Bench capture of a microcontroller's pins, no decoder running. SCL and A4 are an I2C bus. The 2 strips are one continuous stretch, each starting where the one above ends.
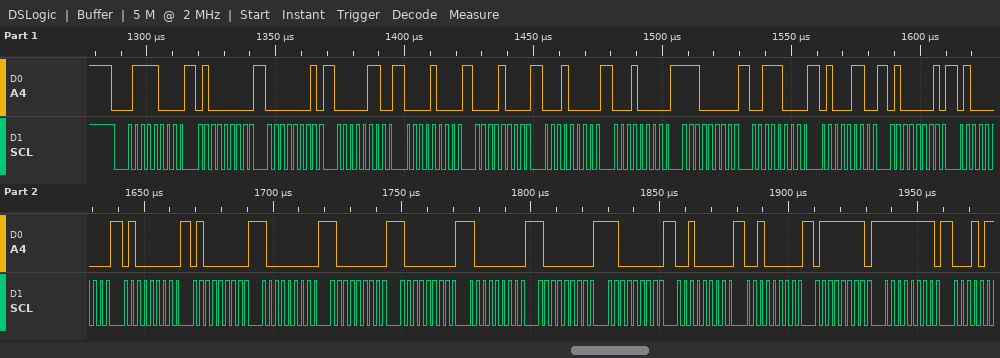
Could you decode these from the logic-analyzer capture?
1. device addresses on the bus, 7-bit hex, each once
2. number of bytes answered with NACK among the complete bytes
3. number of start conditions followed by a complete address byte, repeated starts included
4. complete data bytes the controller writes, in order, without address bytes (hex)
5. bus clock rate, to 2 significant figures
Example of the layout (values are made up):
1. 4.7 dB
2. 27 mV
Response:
1. 0x3C
2. 0
3. 1
4. 40 01 06 08 08 10 10 E0 38 46 41 40 40 40 80 80 80 80 80 C0 20 20 7F FF
5. 400 kHz
